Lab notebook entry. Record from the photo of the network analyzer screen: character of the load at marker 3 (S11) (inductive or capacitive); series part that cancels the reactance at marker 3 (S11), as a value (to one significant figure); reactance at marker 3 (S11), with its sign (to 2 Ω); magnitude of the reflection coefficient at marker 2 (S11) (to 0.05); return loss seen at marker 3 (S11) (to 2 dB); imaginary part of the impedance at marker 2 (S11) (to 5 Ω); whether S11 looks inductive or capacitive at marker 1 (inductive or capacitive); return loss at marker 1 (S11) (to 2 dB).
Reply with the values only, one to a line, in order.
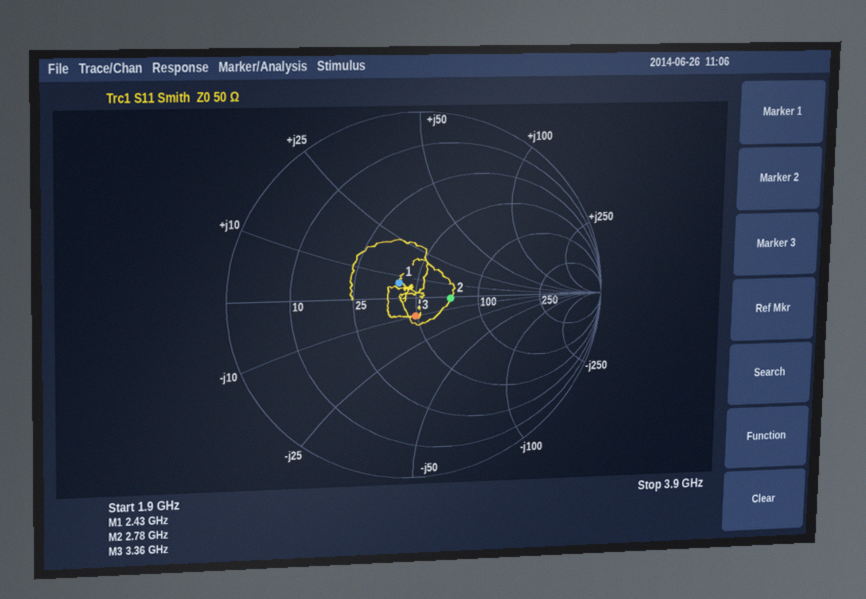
capacitive
500 pH
-10 Ω
0.20
20 dB
0 Ω
inductive
18 dB
